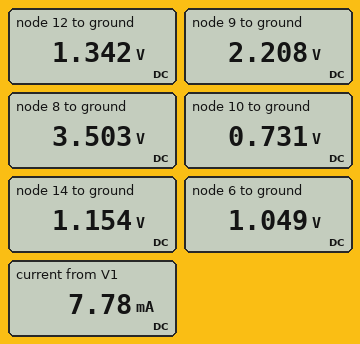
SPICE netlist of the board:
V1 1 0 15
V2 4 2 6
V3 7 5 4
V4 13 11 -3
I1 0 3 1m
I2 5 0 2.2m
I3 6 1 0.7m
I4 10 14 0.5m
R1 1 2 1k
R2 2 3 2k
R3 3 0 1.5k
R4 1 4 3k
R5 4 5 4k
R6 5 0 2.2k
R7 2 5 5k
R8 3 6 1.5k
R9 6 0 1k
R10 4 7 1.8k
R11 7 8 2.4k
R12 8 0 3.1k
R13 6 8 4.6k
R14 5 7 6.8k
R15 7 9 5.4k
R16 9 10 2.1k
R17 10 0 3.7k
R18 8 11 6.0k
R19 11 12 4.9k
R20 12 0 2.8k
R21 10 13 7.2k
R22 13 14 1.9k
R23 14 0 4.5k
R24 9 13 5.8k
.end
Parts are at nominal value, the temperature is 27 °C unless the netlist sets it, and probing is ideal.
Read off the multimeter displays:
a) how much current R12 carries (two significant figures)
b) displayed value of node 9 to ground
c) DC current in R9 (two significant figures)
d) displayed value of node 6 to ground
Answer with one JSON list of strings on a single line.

["1.1 mA", "2.208 V", "1.0 mA", "1.049 V"]
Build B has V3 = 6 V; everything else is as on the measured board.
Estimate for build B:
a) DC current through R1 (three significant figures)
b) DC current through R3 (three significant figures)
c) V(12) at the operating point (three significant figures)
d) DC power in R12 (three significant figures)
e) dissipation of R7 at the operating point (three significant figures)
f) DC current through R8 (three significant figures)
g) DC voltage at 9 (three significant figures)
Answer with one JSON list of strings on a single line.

["7.81 mA", "1.94 mA", "1.43 V", "4.99 mW", "4.50 mW", "1.20 mA", "2.64 V"]
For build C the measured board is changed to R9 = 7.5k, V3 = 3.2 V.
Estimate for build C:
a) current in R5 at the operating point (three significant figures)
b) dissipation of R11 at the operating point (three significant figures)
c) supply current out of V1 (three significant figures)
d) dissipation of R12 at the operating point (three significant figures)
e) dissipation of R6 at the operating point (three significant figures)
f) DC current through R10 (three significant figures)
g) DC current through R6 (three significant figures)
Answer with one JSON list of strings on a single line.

["2.33 mA", "5.11 mW", "7.63 mA", "4.28 mW", "7.07 mW", "3.39 mA", "1.79 mA"]
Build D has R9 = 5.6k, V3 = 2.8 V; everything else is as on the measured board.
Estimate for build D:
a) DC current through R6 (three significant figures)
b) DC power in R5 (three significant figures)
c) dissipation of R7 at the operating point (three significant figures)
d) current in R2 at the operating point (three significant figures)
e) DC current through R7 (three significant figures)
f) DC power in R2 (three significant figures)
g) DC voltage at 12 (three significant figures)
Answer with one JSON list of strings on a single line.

["1.87 mA", "20.7 mW", "1.93 mW", "1.97 mA", "621 µA", "7.75 mW", "1.32 V"]
